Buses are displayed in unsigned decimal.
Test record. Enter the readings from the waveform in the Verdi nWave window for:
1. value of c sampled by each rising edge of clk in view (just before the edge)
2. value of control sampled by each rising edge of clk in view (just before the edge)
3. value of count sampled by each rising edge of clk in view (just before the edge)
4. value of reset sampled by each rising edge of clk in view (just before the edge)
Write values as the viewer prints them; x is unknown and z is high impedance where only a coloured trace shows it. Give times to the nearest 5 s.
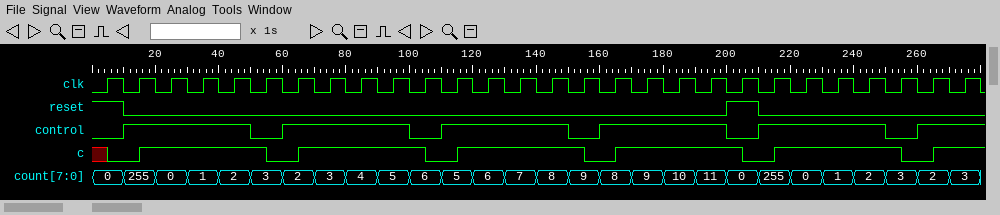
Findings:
x 0 1 1 1 1 0 1 1 1 1 0 1 1 1 1 0 1 1 1 1 0 1 1 1 1 0 1
0 1 1 1 1 0 1 1 1 1 0 1 1 1 1 0 1 1 1 1 0 1 1 1 1 0 1 1
0, 255, 0, 1, 2, 3, 2, 3, 4, 5, 6, 5, 6, 7, 8, 9, 8, 9, 10, 11, 0, 255, 0, 1, 2, 3, 2, 3
1 0 0 0 0 0 0 0 0 0 0 0 0 0 0 0 0 0 0 0 1 0 0 0 0 0 0 0
